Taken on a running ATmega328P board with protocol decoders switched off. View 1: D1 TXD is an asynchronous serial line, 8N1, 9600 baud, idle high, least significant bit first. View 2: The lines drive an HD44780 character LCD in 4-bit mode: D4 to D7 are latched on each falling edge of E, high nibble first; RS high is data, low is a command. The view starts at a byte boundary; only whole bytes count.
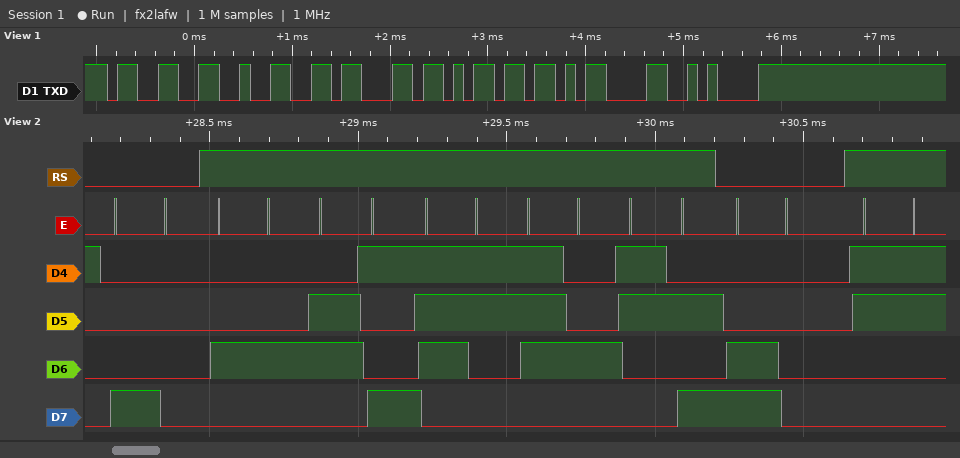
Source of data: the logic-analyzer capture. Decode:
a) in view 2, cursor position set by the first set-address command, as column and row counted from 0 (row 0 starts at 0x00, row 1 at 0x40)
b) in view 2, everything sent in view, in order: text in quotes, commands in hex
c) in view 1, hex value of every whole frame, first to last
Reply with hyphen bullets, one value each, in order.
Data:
- column 0, row 0
- 0x80 "Dist:" 0xC0 "3"
- 33 32 63 6D 0D 0A
